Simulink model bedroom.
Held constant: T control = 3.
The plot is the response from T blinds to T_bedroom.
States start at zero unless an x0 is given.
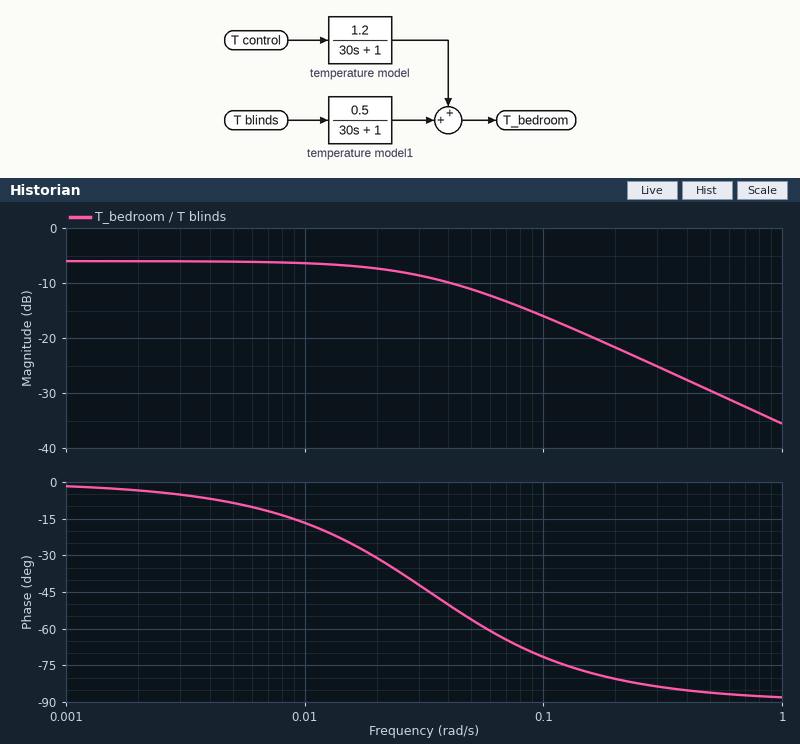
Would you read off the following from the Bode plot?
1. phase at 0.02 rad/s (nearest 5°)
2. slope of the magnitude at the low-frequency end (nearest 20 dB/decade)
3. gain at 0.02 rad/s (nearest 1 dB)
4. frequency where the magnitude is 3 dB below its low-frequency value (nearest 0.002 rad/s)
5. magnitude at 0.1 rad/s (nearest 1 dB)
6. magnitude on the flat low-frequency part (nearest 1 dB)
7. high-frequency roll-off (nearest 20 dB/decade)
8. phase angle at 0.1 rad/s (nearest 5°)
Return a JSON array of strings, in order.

["-30°", "0 dB/decade", "-7 dB", "0.034 rad/s", "-16 dB", "-6 dB", "-20 dB/decade", "-70°"]
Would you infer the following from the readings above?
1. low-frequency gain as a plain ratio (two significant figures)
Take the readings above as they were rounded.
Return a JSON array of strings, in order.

["0.50"]
